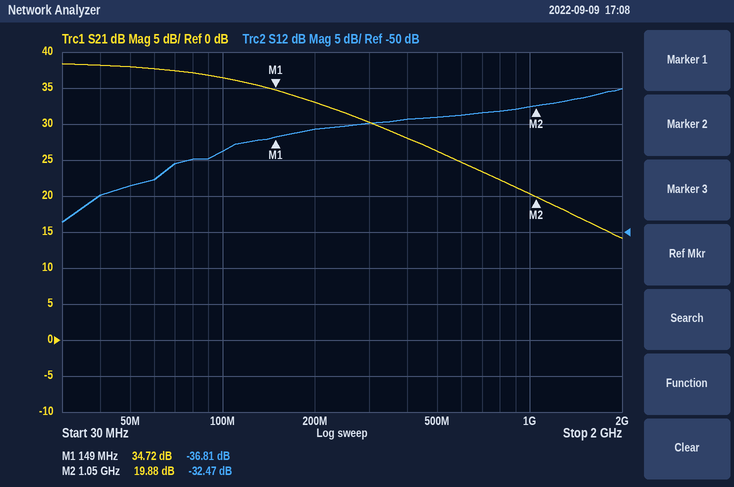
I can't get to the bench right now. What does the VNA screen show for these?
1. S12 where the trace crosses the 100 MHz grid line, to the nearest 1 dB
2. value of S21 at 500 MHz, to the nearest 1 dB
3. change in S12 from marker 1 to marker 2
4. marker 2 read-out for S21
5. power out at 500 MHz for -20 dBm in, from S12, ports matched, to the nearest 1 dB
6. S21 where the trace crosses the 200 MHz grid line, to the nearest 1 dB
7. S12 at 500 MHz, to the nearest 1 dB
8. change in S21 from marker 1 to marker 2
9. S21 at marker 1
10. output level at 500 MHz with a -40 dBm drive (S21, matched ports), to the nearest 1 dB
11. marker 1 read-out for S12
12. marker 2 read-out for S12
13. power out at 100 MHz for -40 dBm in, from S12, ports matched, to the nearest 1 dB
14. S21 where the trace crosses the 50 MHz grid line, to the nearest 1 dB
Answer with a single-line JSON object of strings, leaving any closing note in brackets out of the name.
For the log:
{"S12 where the trace crosses the 100 MHz grid line, to the nearest 1 dB": "-39 dB", "value of S21 at 500 MHz, to the nearest 1 dB": "26 dB", "change in S12 from marker 1 to marker 2": "4.34 dB", "marker 2 read-out for S21": "19.88 dB", "power out at 500 MHz for -20 dBm in, from S12, ports matched, to the nearest 1 dB": "-54 dBm", "S21 where the trace crosses the 200 MHz grid line, to the nearest 1 dB": "33 dB", "S12 at 500 MHz, to the nearest 1 dB": "-34 dB", "change in S21 from marker 1 to marker 2": "-14.84 dB", "S21 at marker 1": "34.72 dB", "output level at 500 MHz with a -40 dBm drive (S21, matched ports), to the nearest 1 dB": "-14 dBm", "marker 1 read-out for S12": "-36.81 dB", "marker 2 read-out for S12": "-32.47 dB", "power out at 100 MHz for -40 dBm in, from S12, ports matched, to the nearest 1 dB": "-79 dBm", "S21 where the trace crosses the 50 MHz grid line, to the nearest 1 dB": "38 dB"}
